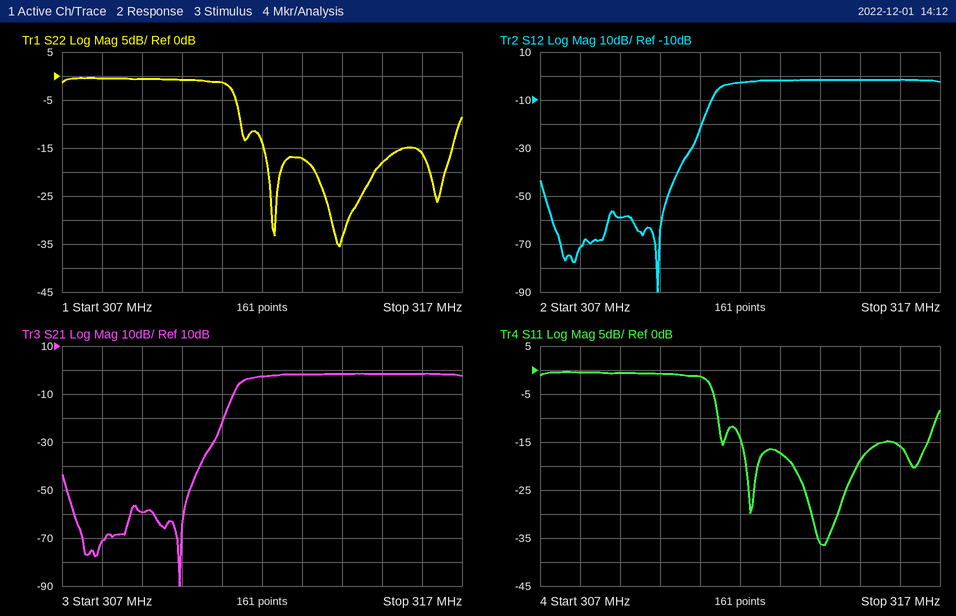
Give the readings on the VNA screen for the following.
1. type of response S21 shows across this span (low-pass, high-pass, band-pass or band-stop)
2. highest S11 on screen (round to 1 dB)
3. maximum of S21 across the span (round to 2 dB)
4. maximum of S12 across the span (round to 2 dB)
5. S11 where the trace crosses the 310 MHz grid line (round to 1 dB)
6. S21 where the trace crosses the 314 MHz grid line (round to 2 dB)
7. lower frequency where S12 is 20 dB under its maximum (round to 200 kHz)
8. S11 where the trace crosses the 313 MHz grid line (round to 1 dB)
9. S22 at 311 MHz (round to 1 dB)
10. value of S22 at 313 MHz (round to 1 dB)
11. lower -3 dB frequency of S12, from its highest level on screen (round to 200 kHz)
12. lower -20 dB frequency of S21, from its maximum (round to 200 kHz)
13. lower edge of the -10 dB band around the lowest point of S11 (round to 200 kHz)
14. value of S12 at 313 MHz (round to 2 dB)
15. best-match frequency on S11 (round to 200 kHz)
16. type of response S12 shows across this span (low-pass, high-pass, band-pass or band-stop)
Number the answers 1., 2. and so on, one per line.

1. high-pass
2. 0 dB
3. -2 dB
4. -2 dB
5. -1 dB
6. -2 dB
7. 311.0 MHz
8. -17 dB
9. -1 dB
10. -17 dB
11. 311.6 MHz
12. 311.0 MHz
13. 311.4 MHz
14. -2 dB
15. 314.0 MHz
16. high-pass
